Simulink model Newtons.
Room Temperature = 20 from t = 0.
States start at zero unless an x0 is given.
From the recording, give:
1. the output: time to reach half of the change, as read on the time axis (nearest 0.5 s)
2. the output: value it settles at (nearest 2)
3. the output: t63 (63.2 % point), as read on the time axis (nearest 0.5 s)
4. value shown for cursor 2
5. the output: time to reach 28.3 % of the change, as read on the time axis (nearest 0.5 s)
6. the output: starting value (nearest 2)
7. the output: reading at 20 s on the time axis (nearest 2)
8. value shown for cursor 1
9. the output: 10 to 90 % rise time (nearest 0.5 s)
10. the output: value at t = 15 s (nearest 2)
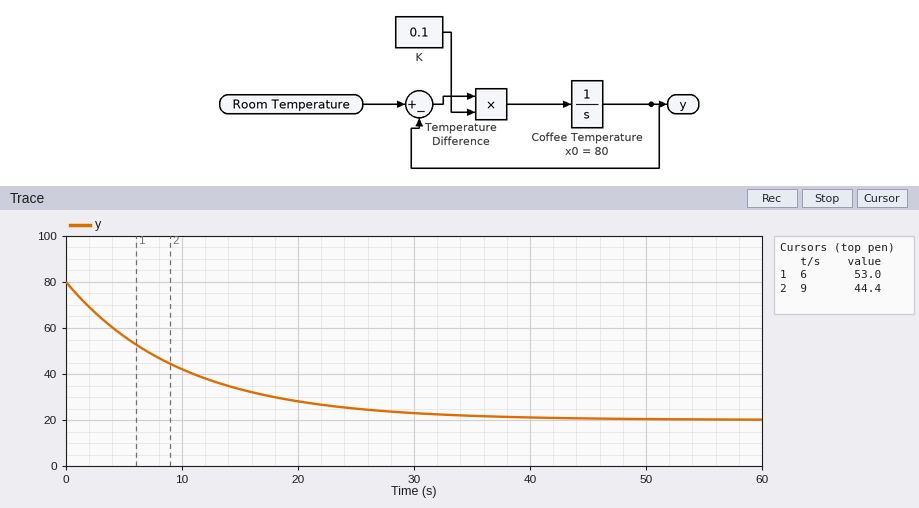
7.0 s
20
10.0 s
44.4
3.5 s
80
28
53.0
22.0 s
34
